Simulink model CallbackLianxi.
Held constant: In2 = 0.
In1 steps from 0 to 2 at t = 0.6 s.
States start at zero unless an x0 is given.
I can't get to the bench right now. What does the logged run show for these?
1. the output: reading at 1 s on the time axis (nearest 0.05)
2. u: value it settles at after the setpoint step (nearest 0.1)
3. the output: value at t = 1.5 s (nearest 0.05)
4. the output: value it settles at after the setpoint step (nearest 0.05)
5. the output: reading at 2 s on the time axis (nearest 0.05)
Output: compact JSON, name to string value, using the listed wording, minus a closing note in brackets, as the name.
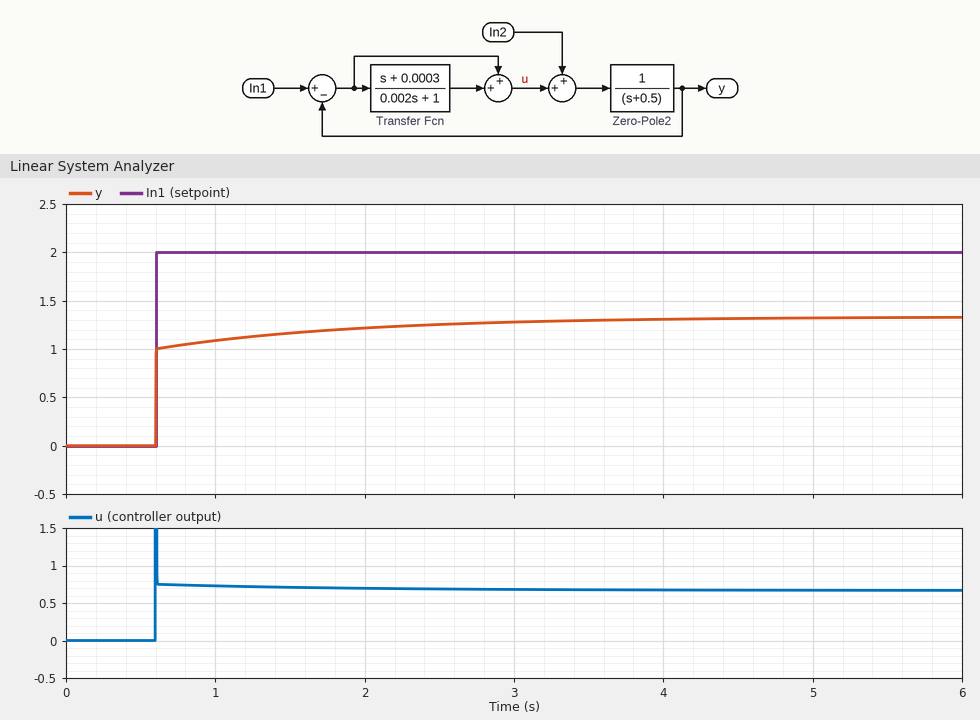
{"the output: reading at 1 s on the time axis": "1.10", "u: value it settles at after the setpoint step": "0.7", "the output: value at t = 1.5 s": "1.15", "the output: value it settles at after the setpoint step": "1.35", "the output: reading at 2 s on the time axis": "1.20"}
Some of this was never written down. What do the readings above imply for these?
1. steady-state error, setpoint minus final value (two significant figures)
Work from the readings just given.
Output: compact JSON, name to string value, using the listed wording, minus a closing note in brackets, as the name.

{"steady-state error, setpoint minus final value": "0.65"}
